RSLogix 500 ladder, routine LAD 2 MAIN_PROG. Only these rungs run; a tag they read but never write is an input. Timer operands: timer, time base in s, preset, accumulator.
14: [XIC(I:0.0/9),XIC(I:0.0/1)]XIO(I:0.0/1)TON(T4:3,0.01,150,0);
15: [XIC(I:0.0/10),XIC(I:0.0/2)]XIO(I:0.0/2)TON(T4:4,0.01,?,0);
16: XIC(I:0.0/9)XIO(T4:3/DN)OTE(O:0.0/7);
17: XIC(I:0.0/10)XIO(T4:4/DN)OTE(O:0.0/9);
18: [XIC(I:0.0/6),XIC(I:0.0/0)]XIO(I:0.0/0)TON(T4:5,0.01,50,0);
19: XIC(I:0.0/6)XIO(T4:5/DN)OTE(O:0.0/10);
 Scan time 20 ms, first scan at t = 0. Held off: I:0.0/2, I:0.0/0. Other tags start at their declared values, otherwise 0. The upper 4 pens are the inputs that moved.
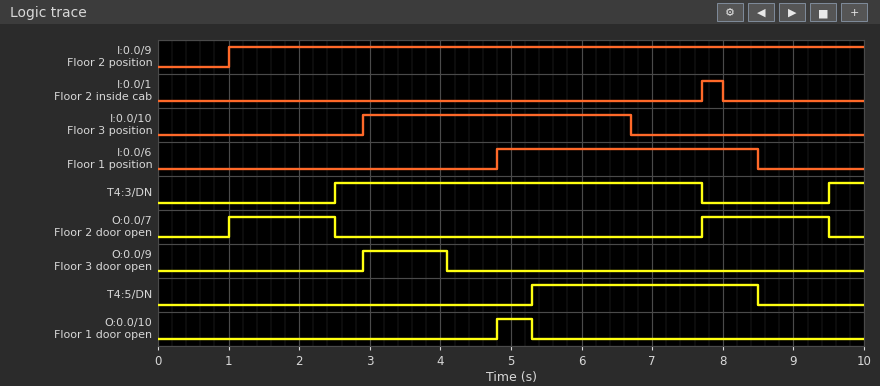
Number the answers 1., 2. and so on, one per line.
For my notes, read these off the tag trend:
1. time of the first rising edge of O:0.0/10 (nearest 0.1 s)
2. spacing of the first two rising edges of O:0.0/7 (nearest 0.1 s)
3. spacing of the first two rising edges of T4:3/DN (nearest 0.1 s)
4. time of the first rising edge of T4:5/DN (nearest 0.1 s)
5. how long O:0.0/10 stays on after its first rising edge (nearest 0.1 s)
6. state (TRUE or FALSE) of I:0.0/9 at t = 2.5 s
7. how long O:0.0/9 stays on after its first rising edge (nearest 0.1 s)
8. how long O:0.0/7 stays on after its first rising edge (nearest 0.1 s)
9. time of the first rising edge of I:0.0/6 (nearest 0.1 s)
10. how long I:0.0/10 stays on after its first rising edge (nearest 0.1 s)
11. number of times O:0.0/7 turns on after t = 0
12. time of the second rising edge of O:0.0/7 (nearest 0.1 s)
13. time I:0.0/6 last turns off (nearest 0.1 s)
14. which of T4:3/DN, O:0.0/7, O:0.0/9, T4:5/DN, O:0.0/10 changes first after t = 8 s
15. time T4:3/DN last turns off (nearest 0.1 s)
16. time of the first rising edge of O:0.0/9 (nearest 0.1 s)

1. 4.8 s
2. 6.7 s
3. 7.0 s
4. 5.3 s
5. 0.5 s
6. TRUE
7. 1.2 s
8. 1.5 s
9. 4.8 s
10. 3.8 s
11. 2
12. 7.7 s
13. 8.5 s
14. T4:5/DN
15. 7.7 s
16. 2.9 s
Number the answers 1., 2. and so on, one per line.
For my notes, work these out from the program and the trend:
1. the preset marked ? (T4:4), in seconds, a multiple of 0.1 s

1. 1.2 s
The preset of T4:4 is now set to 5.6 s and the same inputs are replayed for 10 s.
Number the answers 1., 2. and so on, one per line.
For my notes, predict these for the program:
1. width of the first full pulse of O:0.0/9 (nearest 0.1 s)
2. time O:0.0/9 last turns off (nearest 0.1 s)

1. 3.8 s
2. 6.7 s
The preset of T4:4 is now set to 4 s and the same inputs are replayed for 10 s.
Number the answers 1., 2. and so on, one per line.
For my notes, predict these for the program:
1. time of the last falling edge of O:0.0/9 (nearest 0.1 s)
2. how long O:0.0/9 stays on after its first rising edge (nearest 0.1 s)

1. 6.7 s
2. 3.8 s
